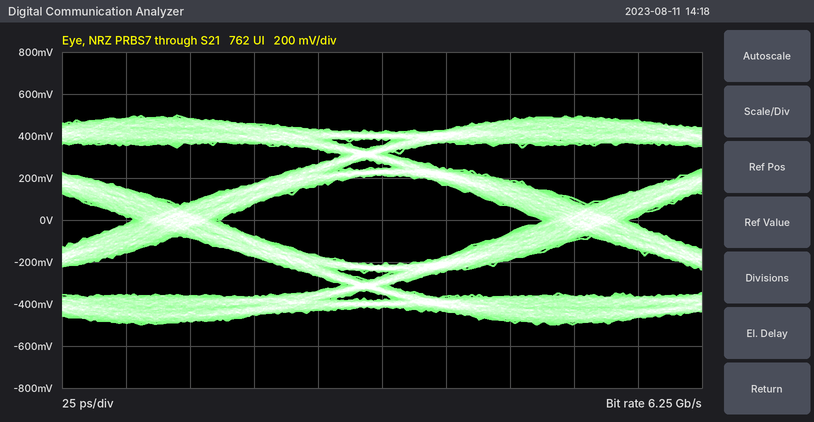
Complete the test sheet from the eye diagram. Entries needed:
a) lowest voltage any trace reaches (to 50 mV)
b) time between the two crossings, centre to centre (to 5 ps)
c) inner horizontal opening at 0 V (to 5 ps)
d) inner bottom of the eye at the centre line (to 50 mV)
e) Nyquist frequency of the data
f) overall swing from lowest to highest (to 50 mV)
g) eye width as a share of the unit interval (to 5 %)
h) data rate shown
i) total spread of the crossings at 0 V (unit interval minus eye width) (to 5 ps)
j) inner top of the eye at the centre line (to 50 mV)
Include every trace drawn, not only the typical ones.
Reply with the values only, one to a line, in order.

-500 mV
160 ps
125 ps
-200 mV
3.125 GHz
1.00 V
80 %
6.25 Gb/s
35 ps
200 mV
